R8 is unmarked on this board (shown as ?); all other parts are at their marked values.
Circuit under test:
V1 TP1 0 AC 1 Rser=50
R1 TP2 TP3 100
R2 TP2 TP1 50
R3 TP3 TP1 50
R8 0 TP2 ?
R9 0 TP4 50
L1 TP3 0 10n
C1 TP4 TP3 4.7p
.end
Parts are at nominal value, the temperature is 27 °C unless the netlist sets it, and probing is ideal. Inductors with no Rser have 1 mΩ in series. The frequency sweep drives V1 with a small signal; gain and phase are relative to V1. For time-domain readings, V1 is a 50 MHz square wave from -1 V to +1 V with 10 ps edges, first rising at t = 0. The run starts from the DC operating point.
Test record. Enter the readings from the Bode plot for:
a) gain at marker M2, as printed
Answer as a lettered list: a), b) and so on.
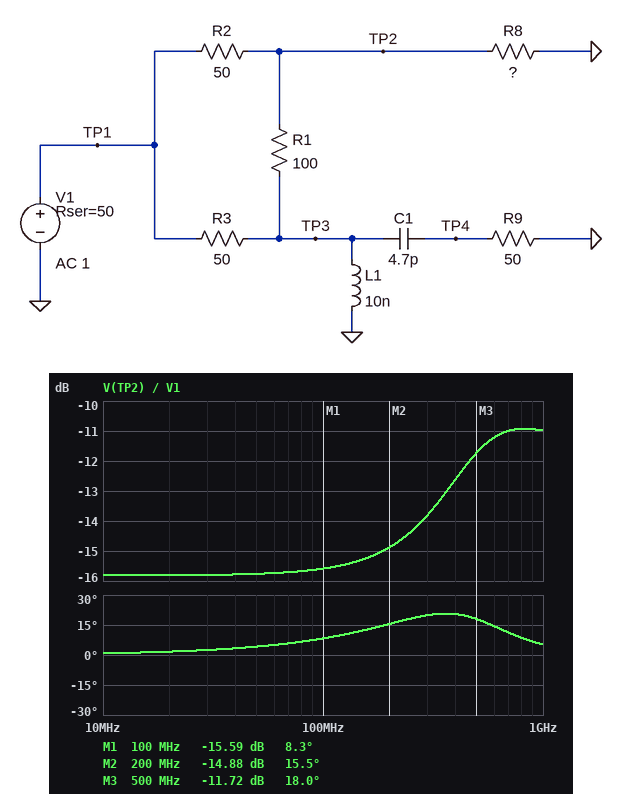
a) -14.88 dB
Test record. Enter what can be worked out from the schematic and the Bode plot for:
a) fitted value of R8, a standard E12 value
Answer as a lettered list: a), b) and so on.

a) 56 Ω
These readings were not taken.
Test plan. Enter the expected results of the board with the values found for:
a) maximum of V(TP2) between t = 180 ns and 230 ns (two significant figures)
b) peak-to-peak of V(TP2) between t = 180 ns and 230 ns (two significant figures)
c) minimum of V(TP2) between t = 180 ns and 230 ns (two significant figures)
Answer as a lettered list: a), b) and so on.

a) 370 mV
b) 740 mV
c) -370 mV
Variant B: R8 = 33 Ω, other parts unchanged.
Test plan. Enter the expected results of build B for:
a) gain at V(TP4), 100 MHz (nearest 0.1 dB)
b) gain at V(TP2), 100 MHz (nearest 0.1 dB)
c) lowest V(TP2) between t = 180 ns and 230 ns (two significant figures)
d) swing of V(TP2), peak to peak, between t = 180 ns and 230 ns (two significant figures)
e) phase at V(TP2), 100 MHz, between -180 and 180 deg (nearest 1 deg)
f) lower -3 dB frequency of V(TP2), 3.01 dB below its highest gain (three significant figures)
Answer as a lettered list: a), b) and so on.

a) -41.8 dB
b) -17.9 dB
c) -270 mV
d) 530 mV
e) 8 deg
f) 258 MHz
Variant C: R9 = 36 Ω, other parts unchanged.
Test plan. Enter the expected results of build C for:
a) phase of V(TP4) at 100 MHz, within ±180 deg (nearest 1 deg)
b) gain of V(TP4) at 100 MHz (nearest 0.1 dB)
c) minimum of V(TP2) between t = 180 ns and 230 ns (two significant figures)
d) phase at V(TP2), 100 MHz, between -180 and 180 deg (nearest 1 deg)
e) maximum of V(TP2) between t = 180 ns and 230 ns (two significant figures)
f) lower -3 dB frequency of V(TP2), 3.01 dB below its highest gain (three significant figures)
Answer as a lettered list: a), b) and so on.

a) 168 deg
b) -44.0 dB
c) -340 mV
d) 8 deg
e) 340 mV
f) 306 MHz
